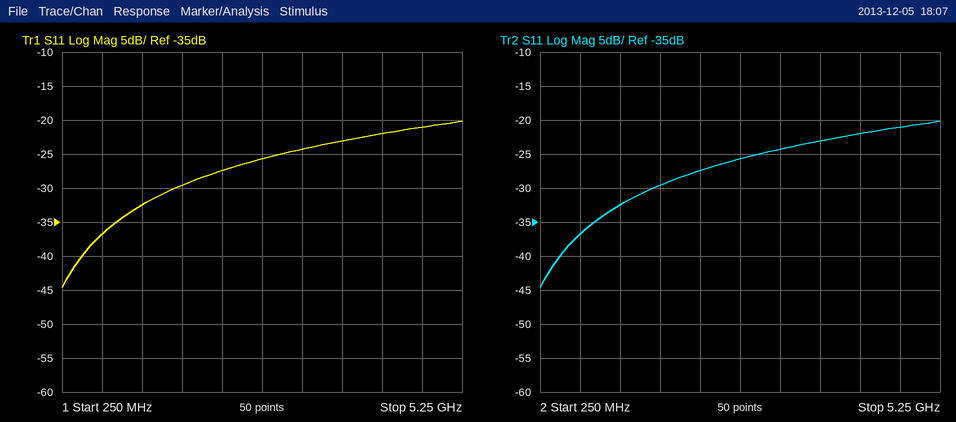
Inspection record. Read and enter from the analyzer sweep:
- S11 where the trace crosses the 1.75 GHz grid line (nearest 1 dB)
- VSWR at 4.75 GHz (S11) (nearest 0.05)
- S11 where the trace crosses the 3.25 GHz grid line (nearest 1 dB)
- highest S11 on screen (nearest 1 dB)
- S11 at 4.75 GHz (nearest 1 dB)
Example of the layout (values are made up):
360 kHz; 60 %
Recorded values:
-30 dB; 1.20; -24 dB; -20 dB; -21 dB
